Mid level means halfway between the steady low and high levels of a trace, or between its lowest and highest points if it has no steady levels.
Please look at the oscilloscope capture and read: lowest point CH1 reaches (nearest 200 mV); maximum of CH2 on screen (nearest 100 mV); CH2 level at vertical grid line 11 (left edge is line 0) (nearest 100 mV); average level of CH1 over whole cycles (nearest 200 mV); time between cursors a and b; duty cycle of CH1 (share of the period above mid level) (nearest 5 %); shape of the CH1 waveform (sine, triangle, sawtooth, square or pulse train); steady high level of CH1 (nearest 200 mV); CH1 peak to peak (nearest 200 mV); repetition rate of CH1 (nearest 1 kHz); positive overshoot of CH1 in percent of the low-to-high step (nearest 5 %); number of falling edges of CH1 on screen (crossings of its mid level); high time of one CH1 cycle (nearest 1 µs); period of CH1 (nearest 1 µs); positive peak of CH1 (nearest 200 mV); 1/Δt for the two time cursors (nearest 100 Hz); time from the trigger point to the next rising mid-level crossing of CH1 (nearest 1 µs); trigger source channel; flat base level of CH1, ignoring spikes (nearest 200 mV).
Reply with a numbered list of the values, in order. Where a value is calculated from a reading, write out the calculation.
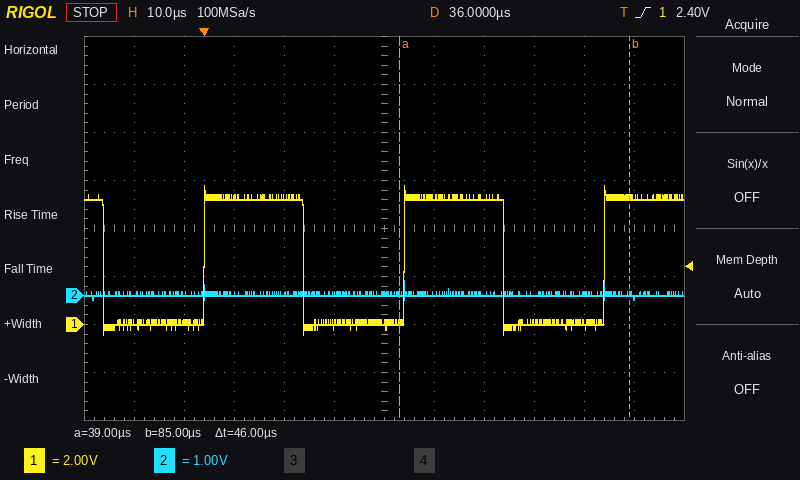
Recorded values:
1. -400 mV
2. 300 mV
3. 0.0 V
4. 0.0 V + 0.5 × (5.2 V − (0.0 V)) ≈ 2.6 V
5. 46 µs
6. 20 µs / 40 µs ≈ 50 %
7. square
8. 5.2 V
9. 5.8 V − (-400 mV) = 6.2 V
10. 1 / 40 µs ≈ 25 kHz
11. 10 %
12. 3
13. 20 µs
14. 40 µs
15. 5.8 V
16. 1 / 46 µs ≈ 21.7 kHz
17. 40 µs
18. CH1
19. 0.0 V
